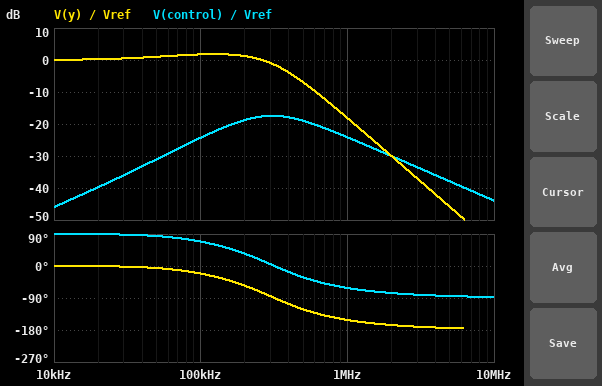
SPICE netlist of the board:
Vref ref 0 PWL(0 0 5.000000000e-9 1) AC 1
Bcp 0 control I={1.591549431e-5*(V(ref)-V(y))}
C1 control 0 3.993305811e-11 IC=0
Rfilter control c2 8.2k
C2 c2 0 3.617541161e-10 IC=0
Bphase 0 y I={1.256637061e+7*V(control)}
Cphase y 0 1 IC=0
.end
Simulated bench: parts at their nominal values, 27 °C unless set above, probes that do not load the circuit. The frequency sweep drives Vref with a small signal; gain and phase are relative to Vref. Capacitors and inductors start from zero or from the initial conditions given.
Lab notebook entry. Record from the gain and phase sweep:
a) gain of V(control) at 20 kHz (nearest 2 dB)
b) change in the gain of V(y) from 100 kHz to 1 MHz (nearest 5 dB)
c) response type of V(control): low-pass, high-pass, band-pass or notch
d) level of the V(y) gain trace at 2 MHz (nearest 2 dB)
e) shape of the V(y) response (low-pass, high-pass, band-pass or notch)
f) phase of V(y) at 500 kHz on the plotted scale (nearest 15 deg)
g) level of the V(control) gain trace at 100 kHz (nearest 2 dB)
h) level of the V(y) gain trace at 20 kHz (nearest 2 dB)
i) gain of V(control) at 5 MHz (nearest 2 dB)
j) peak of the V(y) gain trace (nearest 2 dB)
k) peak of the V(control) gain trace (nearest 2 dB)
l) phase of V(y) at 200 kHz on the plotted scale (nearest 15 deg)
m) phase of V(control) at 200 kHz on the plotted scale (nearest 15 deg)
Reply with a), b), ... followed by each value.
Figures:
a) -40 dB
b) -20 dB
c) band-pass
d) -30 dB
e) low-pass
f) -120 deg
g) -24 dB
h) 0 dB
i) -38 dB
j) 2 dB
k) -18 dB
l) -60 deg
m) 30 deg
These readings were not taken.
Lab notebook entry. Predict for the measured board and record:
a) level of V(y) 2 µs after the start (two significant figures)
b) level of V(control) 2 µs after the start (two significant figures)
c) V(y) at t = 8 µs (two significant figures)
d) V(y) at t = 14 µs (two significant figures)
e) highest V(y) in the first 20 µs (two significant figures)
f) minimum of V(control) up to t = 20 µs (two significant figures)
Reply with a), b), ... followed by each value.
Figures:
a) 1.2 V
b) 2.9 mV
c) 1.0 V
d) 1.0 V
e) 1.2 V
f) -7.4 mV
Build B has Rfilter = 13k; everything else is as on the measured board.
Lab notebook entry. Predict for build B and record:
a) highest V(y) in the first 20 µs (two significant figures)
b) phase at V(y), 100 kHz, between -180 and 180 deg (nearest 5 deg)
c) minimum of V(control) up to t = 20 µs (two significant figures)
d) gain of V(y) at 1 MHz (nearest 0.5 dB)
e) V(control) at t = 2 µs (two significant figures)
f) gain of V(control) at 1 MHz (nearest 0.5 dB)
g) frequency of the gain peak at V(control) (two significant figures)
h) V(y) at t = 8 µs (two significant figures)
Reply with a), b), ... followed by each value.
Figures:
a) 1.3 V
b) -15 deg
c) -24 mV
d) -17.5 dB
e) -21 mV
f) -23.5 dB
g) 340 kHz
h) 1.0 V
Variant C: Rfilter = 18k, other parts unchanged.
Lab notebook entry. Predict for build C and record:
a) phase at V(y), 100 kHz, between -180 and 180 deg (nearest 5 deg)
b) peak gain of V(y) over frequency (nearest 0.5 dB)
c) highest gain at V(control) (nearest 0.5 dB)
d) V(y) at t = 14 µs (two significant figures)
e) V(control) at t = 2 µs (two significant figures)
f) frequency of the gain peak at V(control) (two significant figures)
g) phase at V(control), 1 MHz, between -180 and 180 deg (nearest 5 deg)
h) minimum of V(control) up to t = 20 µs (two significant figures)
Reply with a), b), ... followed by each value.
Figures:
a) -10 deg
b) 5.0 dB
c) -11.0 dB
d) 1.0 V
e) -41 mV
f) 350 kHz
g) -75 deg
h) -43 mV
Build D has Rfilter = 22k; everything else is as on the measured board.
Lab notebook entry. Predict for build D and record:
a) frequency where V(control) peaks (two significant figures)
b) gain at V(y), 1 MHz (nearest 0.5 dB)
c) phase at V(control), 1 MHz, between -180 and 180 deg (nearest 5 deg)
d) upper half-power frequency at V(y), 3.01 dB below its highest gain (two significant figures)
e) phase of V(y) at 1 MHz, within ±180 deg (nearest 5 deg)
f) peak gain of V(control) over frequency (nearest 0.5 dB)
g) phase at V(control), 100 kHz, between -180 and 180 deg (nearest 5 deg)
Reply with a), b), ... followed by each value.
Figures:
a) 350 kHz
b) -17.0 dB
c) -80 deg
d) 410 kHz
e) -170 deg
f) -9.0 dB
g) 80 deg
